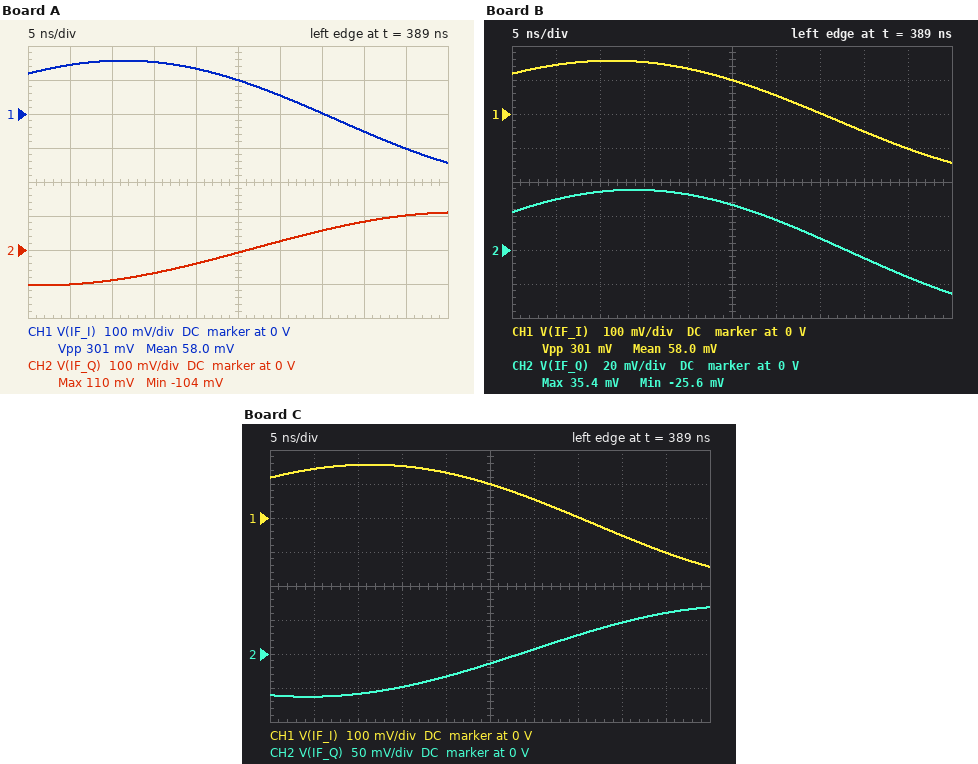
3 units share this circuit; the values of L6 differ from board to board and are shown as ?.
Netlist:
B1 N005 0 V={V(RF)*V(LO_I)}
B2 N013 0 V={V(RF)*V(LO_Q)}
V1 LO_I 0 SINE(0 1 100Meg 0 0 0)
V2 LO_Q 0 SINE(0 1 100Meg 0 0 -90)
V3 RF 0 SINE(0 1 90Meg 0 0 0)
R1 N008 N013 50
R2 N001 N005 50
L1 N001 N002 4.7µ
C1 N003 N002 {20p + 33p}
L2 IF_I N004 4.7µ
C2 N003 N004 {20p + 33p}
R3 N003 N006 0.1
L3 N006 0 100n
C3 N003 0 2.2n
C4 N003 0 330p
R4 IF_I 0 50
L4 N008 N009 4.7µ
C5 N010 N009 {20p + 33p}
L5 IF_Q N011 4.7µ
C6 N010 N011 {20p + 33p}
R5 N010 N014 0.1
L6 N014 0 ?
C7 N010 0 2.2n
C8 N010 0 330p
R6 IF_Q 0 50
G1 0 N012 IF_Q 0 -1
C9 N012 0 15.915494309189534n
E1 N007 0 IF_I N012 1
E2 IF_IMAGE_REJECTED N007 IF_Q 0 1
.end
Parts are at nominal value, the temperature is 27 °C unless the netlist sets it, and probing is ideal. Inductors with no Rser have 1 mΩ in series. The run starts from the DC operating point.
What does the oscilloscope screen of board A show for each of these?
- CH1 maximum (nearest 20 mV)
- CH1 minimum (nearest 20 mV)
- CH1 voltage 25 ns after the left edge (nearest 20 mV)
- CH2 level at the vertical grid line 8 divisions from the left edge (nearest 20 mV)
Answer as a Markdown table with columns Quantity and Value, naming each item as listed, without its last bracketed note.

| Quantity | Value |
|---|---|
| CH1 maximum | 160 mV |
| CH1 minimum | -140 mV |
| CH1 voltage 25 ns after the left edge | 100 mV |
| CH2 level at the vertical grid line 8 divisions from the left edge | 80 mV |
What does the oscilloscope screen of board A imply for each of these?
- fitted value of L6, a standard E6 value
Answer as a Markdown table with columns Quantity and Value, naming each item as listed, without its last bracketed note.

| Quantity | Value |
|---|---|
| fitted value of L6, a standard E6 value | 150 nH |
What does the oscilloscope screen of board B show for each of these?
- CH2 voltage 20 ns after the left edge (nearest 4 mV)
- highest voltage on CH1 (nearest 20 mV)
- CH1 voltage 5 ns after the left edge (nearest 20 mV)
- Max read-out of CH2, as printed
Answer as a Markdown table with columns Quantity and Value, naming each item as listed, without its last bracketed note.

| Quantity | Value |
|---|---|
| CH2 voltage 20 ns after the left edge | 32 mV |
| highest voltage on CH1 | 160 mV |
| CH1 voltage 5 ns after the left edge | 140 mV |
| Max read-out of CH2, as printed | 35.4 mV |
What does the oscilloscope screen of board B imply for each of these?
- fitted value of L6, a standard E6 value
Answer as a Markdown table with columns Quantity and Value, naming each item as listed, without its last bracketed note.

| Quantity | Value |
|---|---|
| fitted value of L6, a standard E6 value | 47 nH |
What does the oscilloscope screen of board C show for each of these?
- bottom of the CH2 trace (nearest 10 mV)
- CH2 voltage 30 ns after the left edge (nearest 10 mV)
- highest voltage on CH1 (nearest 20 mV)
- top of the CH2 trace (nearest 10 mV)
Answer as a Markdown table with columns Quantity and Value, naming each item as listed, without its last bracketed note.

| Quantity | Value |
|---|---|
| bottom of the CH2 trace | -60 mV |
| CH2 voltage 30 ns after the left edge | 10 mV |
| highest voltage on CH1 | 160 mV |
| top of the CH2 trace | 70 mV |
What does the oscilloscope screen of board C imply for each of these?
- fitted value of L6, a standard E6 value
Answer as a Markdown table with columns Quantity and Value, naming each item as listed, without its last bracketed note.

| Quantity | Value |
|---|---|
| fitted value of L6, a standard E6 value | 220 nH |
